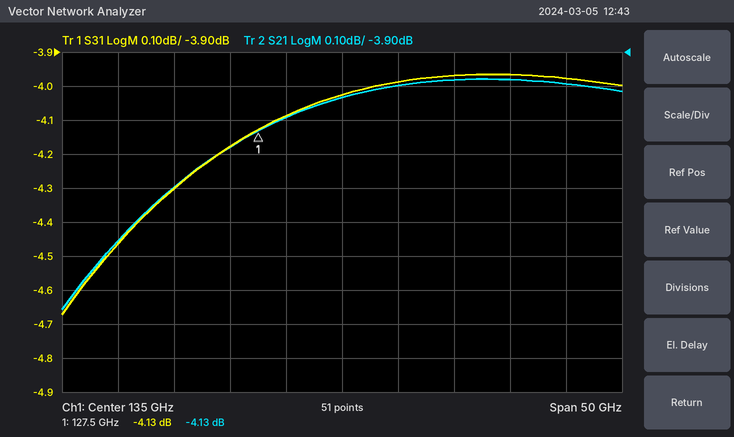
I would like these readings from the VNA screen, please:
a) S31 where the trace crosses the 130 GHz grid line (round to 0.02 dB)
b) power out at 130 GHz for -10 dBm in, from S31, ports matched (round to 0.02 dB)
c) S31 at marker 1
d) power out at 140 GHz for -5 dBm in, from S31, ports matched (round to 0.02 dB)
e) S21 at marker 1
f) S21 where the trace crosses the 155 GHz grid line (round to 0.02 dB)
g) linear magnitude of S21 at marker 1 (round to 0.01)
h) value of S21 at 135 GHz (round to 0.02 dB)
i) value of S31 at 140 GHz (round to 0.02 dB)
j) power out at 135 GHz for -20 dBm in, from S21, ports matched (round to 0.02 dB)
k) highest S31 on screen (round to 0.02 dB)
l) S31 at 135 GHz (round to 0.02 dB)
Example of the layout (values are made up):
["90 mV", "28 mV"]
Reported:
["-4.08 dB", "-14.08 dBm", "-4.13 dB", "-8.98 dBm", "-4.13 dB", "-4.00 dB", "0.62", "-4.04 dB", "-3.98 dB", "-24.04 dBm", "-3.96 dB", "-4.02 dB"]
